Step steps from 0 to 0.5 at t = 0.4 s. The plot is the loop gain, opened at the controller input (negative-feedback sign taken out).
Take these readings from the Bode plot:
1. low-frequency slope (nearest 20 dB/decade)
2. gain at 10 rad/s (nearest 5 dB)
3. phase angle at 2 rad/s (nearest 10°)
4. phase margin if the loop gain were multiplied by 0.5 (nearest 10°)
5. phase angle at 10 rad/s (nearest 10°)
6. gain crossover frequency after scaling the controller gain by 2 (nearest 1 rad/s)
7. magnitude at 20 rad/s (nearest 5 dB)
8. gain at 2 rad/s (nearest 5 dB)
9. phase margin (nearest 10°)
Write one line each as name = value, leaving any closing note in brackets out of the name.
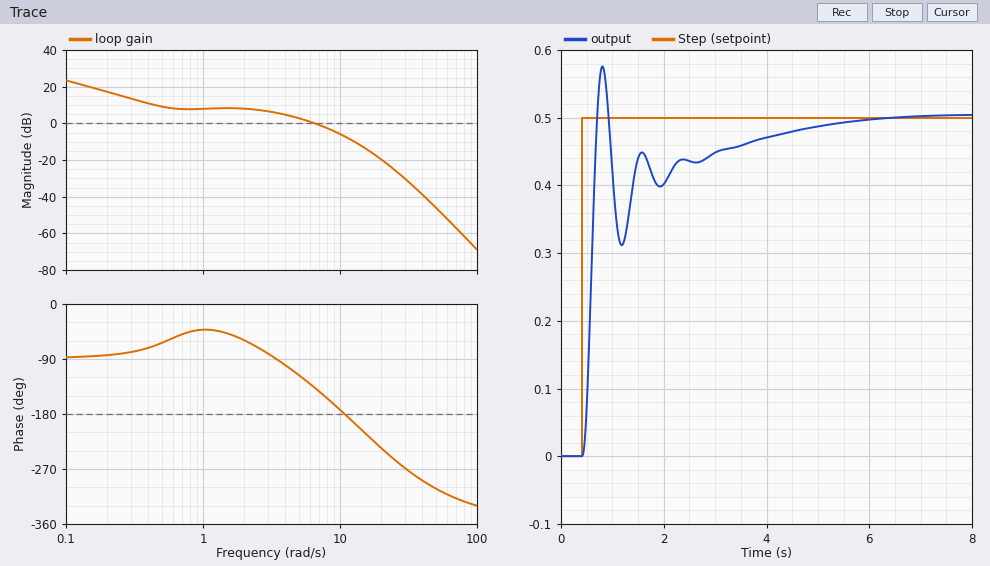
low-frequency slope = -20 dB/decade
gain at 10 rad/s = -5 dB
phase angle at 2 rad/s = -60°
phase margin if the loop gain were multiplied by 0.5 = 90°
phase angle at 10 rad/s = -170°
gain crossover frequency after scaling the controller gain by 2 = 10 rad/s
magnitude at 20 rad/s = -20 dB
gain at 2 rad/s = 10 dB
phase margin = 40°
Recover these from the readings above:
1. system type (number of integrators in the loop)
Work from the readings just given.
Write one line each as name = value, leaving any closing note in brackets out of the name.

system type = 1
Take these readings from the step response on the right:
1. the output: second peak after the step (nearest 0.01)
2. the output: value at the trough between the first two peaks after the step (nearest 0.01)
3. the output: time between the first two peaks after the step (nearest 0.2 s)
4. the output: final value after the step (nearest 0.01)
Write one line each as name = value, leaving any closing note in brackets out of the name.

the output: second peak after the step = 0.45
the output: value at the trough between the first two peaks after the step = 0.31
the output: time between the first two peaks after the step = 0.8 s
the output: final value after the step = 0.50
